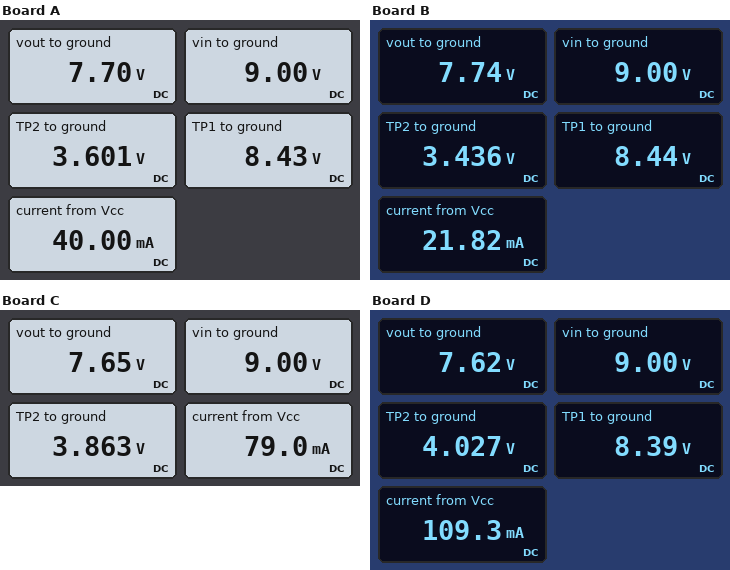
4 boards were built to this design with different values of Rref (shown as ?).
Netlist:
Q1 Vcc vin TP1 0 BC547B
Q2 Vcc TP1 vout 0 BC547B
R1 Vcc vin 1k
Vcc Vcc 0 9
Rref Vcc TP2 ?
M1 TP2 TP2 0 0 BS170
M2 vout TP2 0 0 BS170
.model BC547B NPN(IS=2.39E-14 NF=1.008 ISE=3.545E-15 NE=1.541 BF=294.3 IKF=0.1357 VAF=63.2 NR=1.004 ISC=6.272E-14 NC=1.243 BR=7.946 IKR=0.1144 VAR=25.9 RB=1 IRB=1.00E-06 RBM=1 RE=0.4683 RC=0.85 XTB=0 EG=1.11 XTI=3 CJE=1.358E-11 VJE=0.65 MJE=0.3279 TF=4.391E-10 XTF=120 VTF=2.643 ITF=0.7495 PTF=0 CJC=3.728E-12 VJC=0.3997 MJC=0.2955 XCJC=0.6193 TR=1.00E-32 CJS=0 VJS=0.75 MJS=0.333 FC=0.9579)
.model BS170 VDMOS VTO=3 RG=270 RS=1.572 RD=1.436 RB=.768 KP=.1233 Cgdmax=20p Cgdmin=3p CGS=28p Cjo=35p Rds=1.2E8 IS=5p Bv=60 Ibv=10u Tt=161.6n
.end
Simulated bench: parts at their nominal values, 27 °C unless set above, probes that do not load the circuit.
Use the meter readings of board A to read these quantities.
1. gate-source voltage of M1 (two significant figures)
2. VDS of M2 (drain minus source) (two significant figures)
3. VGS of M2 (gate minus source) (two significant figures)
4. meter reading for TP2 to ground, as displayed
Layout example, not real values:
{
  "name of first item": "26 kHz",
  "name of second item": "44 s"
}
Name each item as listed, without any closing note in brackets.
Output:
{
  "gate-source voltage of M1": "3.6 V",
  "VDS of M2 (drain minus source)": "7.7 V",
  "VGS of M2 (gate minus source)": "3.6 V",
  "meter reading for TP2 to ground, as displayed": "3.601 V"
}
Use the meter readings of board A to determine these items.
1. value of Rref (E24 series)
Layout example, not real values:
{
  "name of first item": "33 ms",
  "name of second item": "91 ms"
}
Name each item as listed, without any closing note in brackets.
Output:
{
  "value of Rref": "270 Ω"
}
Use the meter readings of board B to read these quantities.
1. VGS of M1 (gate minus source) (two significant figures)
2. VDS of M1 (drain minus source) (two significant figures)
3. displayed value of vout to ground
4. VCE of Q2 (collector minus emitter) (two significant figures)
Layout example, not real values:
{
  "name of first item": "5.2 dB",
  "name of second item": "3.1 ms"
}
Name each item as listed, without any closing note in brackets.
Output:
{
  "VGS of M1 (gate minus source)": "3.4 V",
  "VDS of M1 (drain minus source)": "3.4 V",
  "displayed value of vout to ground": "7.74 V",
  "VCE of Q2 (collector minus emitter)": "1.3 V"
}
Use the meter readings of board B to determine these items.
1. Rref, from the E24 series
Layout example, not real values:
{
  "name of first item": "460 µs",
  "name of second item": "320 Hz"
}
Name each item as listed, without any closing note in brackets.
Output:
{
  "Rref, from the E24 series": "510 Ω"
}
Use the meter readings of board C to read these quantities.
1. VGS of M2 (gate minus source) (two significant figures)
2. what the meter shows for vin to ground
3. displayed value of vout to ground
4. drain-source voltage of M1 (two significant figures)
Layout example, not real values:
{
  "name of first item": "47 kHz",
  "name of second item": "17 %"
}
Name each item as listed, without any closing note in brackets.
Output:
{
  "VGS of M2 (gate minus source)": "3.9 V",
  "what the meter shows for vin to ground": "9.00 V",
  "displayed value of vout to ground": "7.65 V",
  "drain-source voltage of M1": "3.9 V"
}
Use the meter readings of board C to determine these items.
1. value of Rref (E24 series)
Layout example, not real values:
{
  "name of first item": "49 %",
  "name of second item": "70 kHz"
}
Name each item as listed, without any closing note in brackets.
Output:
{
  "value of Rref": "130 Ω"
}
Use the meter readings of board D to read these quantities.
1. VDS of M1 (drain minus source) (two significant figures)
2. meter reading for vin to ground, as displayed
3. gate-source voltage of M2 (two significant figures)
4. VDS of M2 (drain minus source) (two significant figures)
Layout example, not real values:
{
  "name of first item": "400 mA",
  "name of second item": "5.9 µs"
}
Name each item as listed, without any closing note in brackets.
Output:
{
  "VDS of M1 (drain minus source)": "4.0 V",
  "meter reading for vin to ground, as displayed": "9.00 V",
  "gate-source voltage of M2": "4.0 V",
  "VDS of M2 (drain minus source)": "7.6 V"
}
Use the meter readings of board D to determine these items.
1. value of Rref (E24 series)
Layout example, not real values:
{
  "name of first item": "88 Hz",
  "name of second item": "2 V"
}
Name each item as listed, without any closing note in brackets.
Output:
{
  "value of Rref": "91 Ω"
}
